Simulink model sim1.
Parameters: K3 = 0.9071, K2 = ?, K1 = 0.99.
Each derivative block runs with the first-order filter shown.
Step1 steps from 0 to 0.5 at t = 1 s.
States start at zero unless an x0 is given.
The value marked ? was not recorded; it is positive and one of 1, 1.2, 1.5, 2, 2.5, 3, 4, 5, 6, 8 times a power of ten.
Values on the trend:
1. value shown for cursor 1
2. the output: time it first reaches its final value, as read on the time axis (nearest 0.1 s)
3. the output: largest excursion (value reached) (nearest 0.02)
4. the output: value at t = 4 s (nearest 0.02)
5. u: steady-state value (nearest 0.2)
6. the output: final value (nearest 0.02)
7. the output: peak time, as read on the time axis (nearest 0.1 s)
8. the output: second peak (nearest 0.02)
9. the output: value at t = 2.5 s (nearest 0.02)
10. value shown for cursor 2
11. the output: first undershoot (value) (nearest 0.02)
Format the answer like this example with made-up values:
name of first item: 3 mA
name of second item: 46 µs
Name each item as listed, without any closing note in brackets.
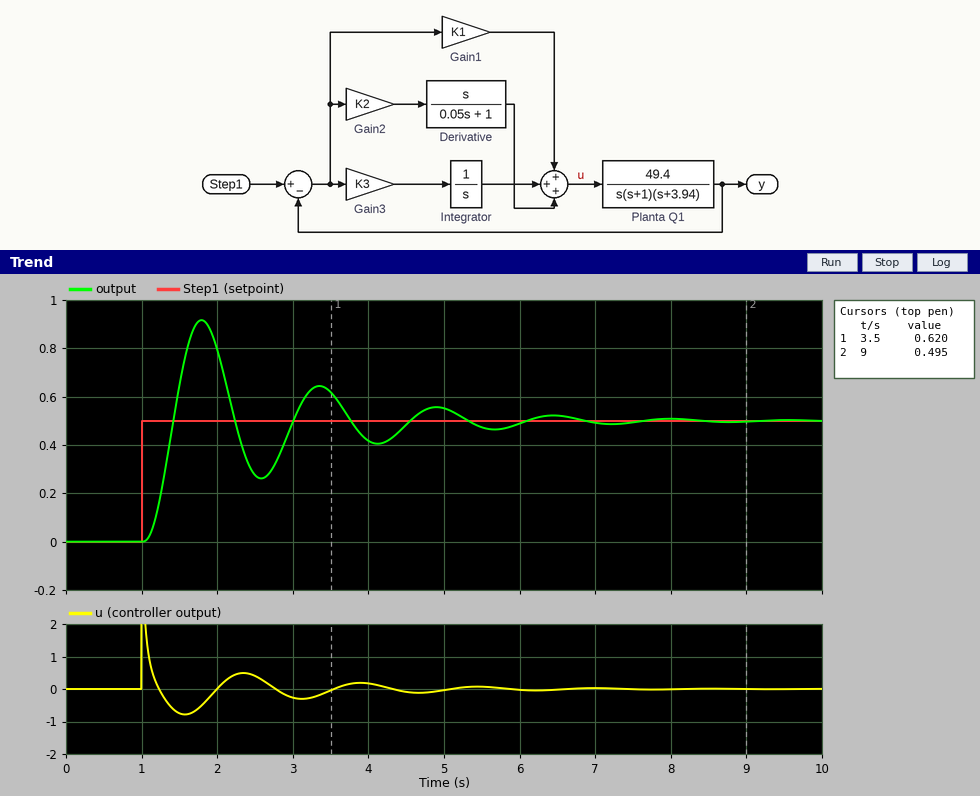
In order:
value shown for cursor 1: 0.620
the output: time it first reaches its final value, as read on the time axis: 1.4 s
the output: largest excursion (value reached): 0.92
the output: value at t = 4 s: 0.42
u: steady-state value: 0.0
the output: final value: 0.50
the output: peak time, as read on the time axis: 1.8 s
the output: second peak: 0.64
the output: value at t = 2.5 s: 0.28
value shown for cursor 2: 0.495
the output: first undershoot (value): 0.26
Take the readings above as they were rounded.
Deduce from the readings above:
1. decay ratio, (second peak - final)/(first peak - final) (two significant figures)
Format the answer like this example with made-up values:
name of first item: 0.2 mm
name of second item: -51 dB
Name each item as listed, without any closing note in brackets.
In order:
decay ratio, (second peak - final)/(first peak - final): 0.33
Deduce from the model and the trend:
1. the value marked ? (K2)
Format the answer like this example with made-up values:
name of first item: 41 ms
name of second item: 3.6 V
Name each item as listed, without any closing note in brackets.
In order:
the value marked ?: 0.4
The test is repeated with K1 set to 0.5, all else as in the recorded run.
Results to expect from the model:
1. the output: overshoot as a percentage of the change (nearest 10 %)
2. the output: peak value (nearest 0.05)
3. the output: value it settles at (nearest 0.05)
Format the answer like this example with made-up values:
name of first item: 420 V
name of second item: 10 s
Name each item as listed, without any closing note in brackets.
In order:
the output: overshoot as a percentage of the change: 60 %
the output: peak value: 0.80
the output: value it settles at: 0.50
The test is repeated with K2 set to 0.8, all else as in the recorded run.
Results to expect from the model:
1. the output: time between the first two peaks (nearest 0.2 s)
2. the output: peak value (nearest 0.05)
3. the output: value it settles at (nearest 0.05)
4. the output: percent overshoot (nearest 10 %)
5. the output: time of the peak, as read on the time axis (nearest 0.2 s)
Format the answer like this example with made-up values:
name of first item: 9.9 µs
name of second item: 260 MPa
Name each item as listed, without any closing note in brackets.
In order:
the output: time between the first two peaks: 1.0 s
the output: peak value: 0.85
the output: value it settles at: 0.50
the output: percent overshoot: 70 %
the output: time of the peak, as read on the time axis: 1.6 s
